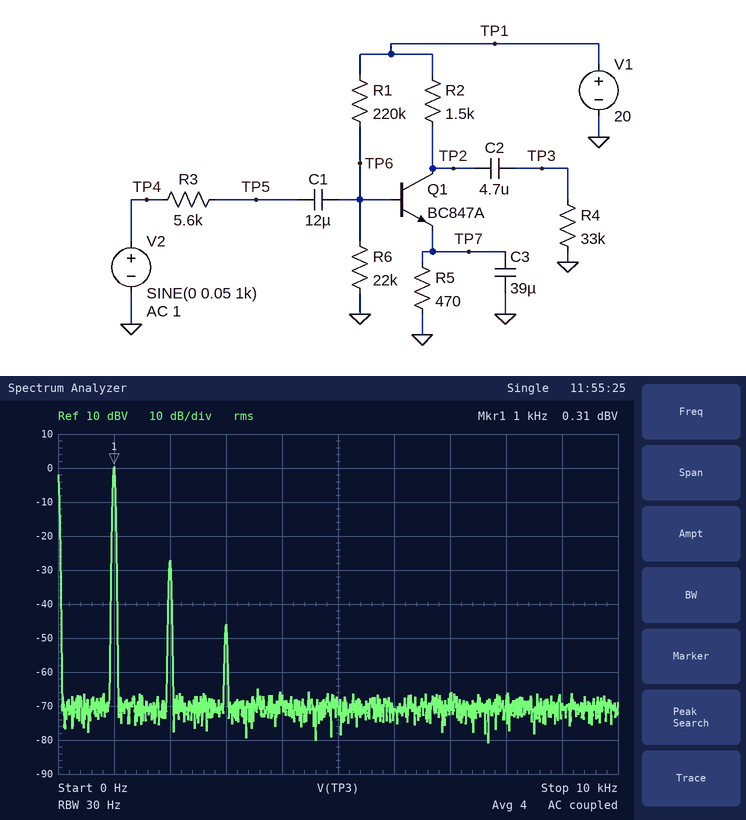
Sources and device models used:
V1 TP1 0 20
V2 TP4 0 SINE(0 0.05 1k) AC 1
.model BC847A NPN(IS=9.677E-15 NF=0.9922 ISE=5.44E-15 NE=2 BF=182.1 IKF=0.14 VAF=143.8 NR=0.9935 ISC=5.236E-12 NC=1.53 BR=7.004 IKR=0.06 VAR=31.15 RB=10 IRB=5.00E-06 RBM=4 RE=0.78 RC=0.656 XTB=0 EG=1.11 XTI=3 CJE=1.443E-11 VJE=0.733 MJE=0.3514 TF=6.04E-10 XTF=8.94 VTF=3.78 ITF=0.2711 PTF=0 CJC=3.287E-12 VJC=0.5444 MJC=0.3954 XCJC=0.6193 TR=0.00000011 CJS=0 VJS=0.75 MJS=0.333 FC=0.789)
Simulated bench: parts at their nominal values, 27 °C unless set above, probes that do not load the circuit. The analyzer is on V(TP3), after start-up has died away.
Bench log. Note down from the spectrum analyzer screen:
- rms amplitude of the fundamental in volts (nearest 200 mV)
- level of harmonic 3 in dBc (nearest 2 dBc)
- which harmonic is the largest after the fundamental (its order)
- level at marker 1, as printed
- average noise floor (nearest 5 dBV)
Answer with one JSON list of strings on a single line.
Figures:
["1.0 V", "-46 dBc", "2", "0.31 dBV", "-70 dBV"]
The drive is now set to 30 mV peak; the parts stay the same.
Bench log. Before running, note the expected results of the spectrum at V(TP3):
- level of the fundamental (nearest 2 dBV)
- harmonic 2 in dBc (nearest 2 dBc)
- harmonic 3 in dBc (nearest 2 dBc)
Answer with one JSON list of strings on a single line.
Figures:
["-4 dBV", "-32 dBc", "-56 dBc"]
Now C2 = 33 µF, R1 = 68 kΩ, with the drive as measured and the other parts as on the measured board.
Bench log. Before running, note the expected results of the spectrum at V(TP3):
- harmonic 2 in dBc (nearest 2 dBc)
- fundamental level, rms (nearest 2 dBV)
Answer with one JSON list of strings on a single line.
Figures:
["-48 dBc", "2 dBV"]
